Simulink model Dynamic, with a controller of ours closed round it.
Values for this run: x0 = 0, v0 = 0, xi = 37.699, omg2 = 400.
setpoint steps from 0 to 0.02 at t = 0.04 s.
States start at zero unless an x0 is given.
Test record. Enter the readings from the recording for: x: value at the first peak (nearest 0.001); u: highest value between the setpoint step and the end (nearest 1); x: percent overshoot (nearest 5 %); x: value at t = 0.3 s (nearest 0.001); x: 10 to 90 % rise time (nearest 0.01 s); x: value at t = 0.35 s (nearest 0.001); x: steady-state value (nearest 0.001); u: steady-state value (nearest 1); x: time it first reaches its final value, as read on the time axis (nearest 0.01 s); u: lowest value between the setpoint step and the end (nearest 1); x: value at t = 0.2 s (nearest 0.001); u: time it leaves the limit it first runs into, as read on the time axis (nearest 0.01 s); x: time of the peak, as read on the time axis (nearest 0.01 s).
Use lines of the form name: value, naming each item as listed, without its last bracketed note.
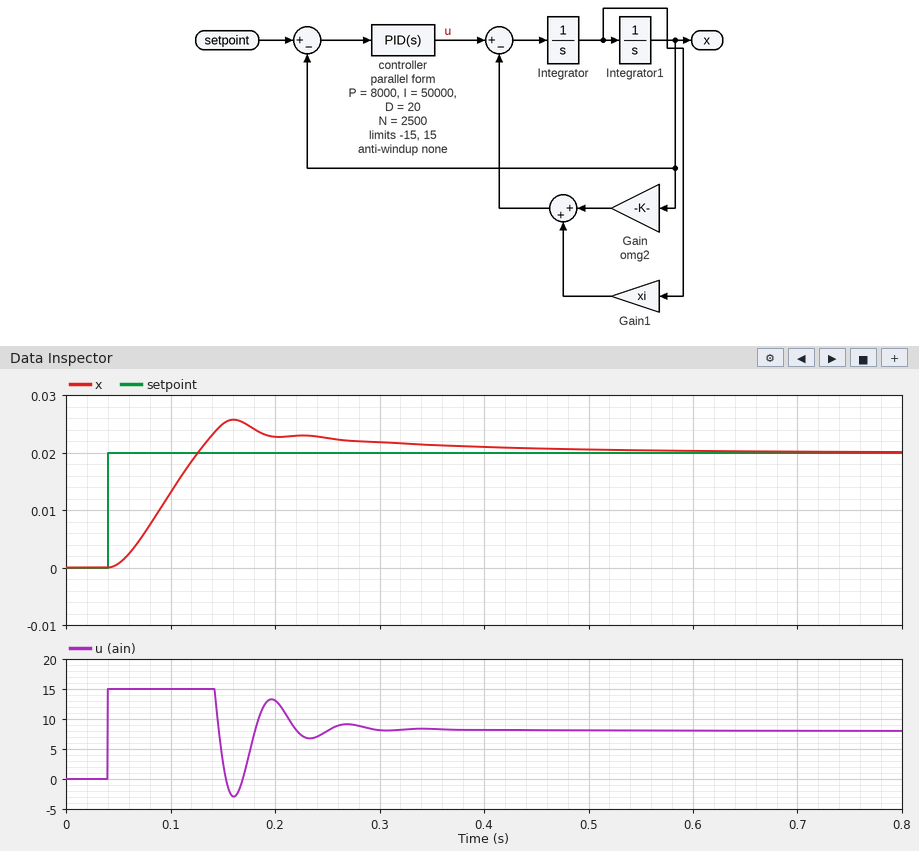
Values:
x: value at the first peak: 0.026
u: highest value between the setpoint step and the end: 15
x: percent overshoot: 30 %
x: value at t = 0.3 s: 0.022
x: 10 to 90 % rise time: 0.06 s
x: value at t = 0.35 s: 0.021
x: steady-state value: 0.020
u: steady-state value: 8
x: time it first reaches its final value, as read on the time axis: 0.13 s
u: lowest value between the setpoint step and the end: -3
x: value at t = 0.2 s: 0.023
u: time it leaves the limit it first runs into, as read on the time axis: 0.14 s
x: time of the peak, as read on the time axis: 0.16 s
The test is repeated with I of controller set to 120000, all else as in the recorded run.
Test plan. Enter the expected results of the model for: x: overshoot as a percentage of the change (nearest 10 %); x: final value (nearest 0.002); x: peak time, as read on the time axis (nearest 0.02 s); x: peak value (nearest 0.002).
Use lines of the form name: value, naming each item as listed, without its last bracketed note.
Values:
x: overshoot as a percentage of the change: 50 %
x: final value: 0.020
x: peak time, as read on the time axis: 0.18 s
x: peak value: 0.030
